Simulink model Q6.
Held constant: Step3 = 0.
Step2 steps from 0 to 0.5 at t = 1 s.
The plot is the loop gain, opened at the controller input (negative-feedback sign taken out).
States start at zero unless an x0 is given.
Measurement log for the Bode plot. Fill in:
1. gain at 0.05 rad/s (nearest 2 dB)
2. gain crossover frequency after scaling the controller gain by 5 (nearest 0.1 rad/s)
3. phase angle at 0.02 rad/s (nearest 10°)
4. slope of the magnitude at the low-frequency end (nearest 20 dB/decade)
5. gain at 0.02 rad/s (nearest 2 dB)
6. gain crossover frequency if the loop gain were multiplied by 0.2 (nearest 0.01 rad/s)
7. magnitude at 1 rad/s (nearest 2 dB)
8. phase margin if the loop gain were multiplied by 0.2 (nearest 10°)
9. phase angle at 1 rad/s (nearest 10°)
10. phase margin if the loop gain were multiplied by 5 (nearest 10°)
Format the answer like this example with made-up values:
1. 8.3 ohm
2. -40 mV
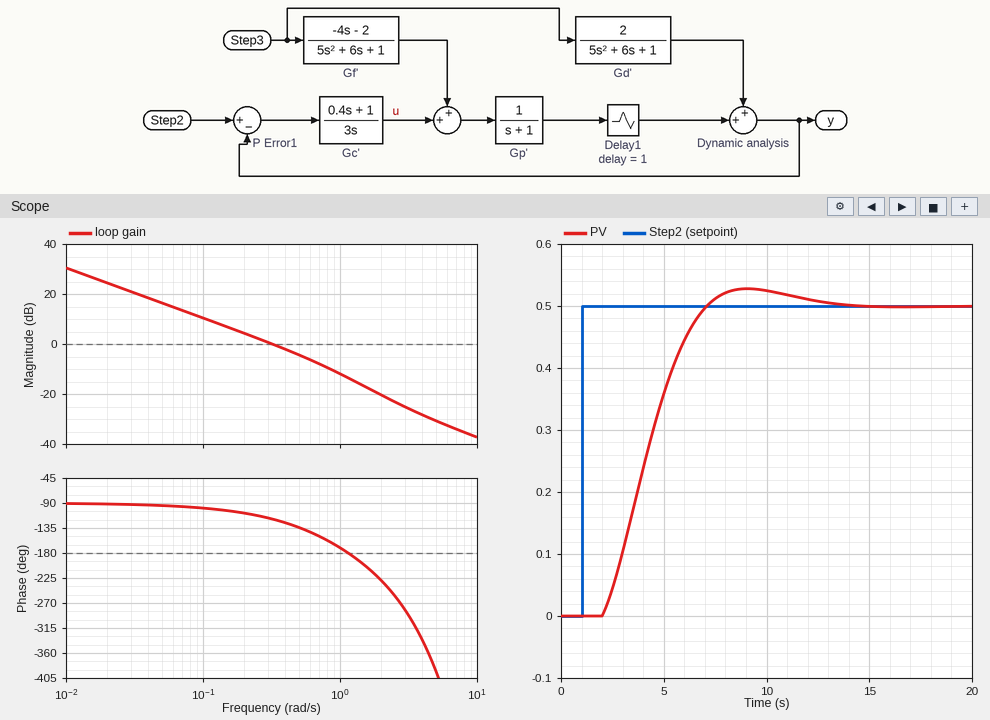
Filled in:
1. 16 dB
2. 1.2 rad/s
3. -90°
4. -20 dB/decade
5. 24 dB
6. 0.07 rad/s
7. -12 dB
8. 80°
9. -170°
10. 0°
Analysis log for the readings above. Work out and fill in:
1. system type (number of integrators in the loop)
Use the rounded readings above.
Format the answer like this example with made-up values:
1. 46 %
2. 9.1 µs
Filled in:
1. 1
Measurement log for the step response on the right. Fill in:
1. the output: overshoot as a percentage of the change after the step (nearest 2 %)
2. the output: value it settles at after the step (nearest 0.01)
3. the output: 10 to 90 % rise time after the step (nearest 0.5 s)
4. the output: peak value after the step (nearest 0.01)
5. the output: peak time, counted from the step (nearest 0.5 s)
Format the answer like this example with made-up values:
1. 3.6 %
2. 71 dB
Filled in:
1. 6 %
2. 0.50
3. 3.5 s
4. 0.53
5. 8.0 s
